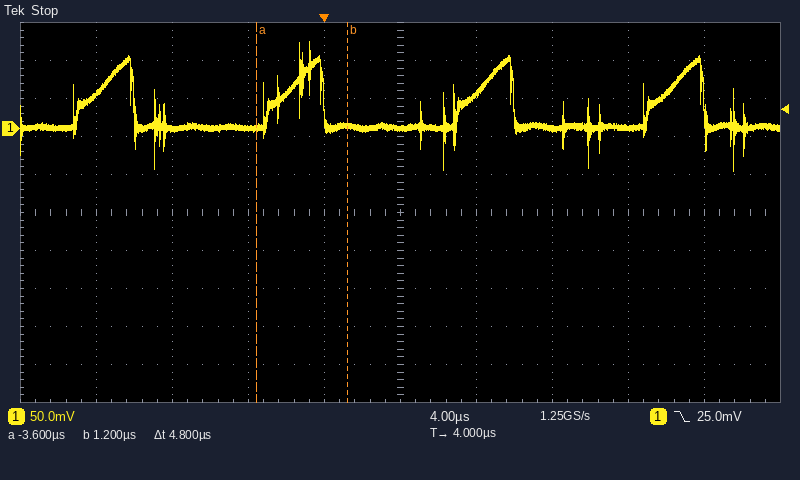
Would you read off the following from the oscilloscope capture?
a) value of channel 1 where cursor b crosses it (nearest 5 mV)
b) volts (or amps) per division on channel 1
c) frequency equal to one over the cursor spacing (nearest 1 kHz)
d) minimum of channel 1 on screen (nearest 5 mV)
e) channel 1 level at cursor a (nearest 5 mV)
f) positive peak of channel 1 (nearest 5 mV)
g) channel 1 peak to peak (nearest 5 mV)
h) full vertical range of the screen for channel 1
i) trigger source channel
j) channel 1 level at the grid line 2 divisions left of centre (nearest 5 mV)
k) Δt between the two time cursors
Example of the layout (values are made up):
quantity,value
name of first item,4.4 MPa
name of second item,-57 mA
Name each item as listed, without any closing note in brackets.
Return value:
quantity,value
value of channel 1 where cursor b crosses it,5 mV
volts (or amps) per division on channel 1,50 mV
frequency equal to one over the cursor spacing,208 kHz
minimum of channel 1 on screen,-55 mV
channel 1 level at cursor a,0 mV
positive peak of channel 1,115 mV
channel 1 peak to peak,170 mV
full vertical range of the screen for channel 1,500 mV
trigger source channel,channel 1
channel 1 level at the grid line 2 divisions left of centre,0 mV
Δt between the two time cursors,4.8 µs
